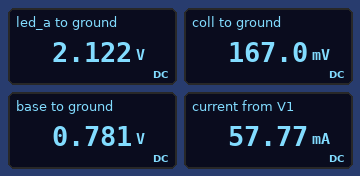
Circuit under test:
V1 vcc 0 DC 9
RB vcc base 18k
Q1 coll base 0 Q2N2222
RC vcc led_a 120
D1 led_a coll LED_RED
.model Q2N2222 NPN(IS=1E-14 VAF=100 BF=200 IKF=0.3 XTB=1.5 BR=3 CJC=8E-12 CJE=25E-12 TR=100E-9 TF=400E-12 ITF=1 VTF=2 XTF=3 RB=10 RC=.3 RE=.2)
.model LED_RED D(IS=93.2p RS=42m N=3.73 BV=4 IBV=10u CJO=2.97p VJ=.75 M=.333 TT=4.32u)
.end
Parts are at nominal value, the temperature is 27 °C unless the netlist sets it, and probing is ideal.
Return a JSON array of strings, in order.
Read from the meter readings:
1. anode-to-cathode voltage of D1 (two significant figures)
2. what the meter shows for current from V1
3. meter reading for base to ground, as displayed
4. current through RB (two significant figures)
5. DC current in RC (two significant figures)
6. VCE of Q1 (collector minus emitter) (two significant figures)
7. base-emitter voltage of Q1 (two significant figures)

["2.0 V", "57.77 mA", "0.781 V", "460 µA", "57 mA", "170 mV", "780 mV"]
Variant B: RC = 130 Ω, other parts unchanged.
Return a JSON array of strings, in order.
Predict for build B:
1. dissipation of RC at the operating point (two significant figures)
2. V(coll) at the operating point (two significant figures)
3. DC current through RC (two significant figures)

["370 mW", "160 mV", "53 mA"]
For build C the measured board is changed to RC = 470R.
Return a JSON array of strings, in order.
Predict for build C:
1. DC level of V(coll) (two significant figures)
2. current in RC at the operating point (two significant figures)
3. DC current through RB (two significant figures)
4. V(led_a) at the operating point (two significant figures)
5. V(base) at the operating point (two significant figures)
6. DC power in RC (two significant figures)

["79 mV", "15 mA", "460 µA", "1.9 V", "740 mV", "110 mW"]
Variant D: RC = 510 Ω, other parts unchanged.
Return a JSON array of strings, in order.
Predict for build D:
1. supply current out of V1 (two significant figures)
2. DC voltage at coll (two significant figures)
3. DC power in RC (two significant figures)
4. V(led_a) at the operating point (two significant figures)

["14 mA", "76 mV", "99 mW", "1.9 V"]
